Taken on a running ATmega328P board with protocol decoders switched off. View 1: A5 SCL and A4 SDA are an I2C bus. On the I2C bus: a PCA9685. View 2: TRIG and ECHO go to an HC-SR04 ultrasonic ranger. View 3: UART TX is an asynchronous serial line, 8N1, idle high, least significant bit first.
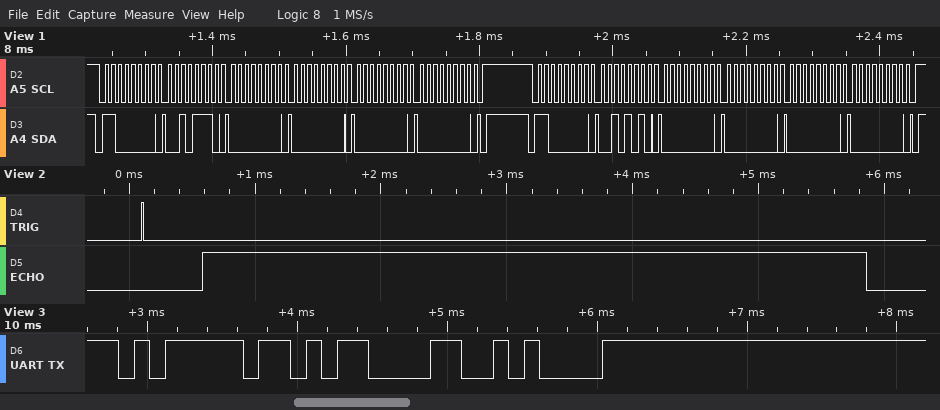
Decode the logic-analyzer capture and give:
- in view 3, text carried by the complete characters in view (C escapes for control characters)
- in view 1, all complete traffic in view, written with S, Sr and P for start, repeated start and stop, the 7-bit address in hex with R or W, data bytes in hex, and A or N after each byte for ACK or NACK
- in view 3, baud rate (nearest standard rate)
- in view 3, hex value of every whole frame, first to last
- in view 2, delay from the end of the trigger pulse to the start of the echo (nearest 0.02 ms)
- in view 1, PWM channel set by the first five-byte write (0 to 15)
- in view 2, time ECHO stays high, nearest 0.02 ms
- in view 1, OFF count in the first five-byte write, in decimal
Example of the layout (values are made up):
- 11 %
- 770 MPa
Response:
- "}\r\n"
- S 60W A 2E A 00 A 00 A 00 A 00 A P S 60W A 2A A 00 A 00 A 00 A 00 A P
- 9600 baud
- 7D 0D 0A
- 0.46 ms
- 10
- 5.28 ms
- 0
